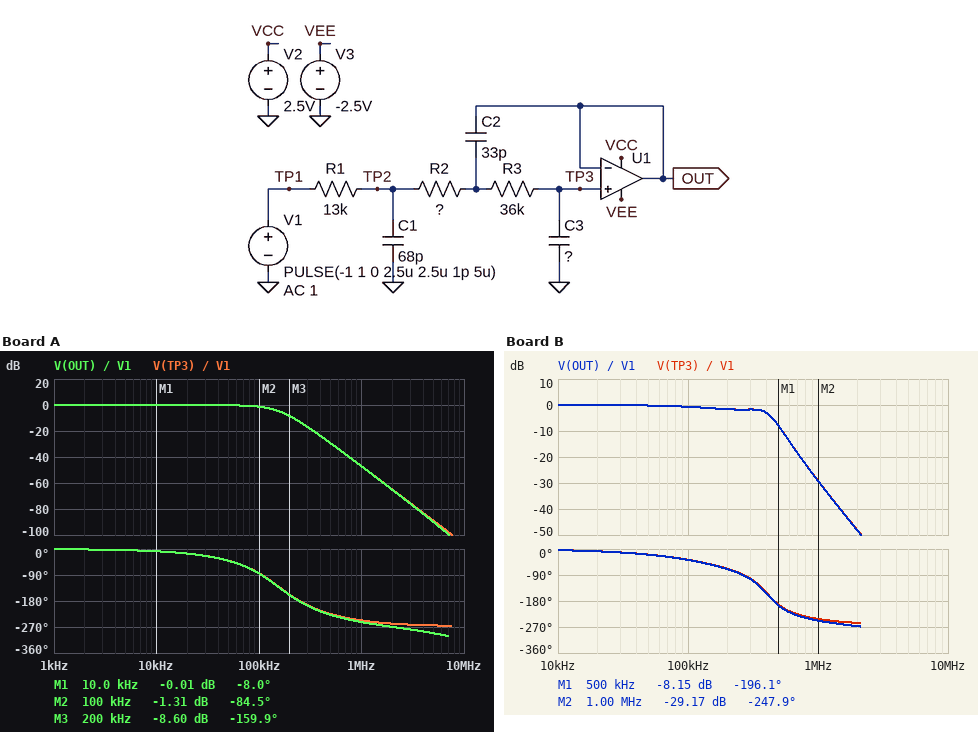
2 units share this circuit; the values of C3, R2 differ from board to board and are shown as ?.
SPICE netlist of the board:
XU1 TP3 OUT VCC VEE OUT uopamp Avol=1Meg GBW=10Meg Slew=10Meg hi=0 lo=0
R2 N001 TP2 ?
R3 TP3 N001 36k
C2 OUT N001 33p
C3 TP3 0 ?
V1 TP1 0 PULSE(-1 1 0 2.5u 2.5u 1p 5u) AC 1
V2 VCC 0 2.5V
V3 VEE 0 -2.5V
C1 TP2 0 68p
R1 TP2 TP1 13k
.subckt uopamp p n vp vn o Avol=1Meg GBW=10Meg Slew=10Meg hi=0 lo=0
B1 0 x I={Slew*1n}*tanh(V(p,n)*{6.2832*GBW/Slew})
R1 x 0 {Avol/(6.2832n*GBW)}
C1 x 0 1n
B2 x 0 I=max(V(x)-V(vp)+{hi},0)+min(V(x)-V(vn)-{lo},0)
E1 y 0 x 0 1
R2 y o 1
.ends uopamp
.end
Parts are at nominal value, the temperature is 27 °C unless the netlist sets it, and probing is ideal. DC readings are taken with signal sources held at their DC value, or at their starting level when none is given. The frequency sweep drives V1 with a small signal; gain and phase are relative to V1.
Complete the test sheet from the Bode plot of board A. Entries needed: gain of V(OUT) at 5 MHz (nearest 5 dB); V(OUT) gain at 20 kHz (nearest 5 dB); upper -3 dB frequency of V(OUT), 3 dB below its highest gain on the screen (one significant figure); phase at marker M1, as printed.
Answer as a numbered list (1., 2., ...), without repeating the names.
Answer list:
1. -90 dB
2. 0 dB
3. 100 kHz
4. -8.0 deg
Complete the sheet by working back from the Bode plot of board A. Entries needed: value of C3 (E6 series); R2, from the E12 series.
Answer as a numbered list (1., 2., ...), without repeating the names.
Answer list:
1. 10 pF
2. 82 kΩ
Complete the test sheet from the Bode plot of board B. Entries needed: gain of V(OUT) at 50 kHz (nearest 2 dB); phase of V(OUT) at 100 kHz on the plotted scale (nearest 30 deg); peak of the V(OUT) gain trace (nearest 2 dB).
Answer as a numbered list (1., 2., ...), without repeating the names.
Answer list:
1. 0 dB
2. -30 deg
3. 0 dB
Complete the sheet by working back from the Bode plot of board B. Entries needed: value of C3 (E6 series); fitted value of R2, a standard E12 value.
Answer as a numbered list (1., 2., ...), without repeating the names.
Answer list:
1. 2.2 pF
2. 47 kΩ
